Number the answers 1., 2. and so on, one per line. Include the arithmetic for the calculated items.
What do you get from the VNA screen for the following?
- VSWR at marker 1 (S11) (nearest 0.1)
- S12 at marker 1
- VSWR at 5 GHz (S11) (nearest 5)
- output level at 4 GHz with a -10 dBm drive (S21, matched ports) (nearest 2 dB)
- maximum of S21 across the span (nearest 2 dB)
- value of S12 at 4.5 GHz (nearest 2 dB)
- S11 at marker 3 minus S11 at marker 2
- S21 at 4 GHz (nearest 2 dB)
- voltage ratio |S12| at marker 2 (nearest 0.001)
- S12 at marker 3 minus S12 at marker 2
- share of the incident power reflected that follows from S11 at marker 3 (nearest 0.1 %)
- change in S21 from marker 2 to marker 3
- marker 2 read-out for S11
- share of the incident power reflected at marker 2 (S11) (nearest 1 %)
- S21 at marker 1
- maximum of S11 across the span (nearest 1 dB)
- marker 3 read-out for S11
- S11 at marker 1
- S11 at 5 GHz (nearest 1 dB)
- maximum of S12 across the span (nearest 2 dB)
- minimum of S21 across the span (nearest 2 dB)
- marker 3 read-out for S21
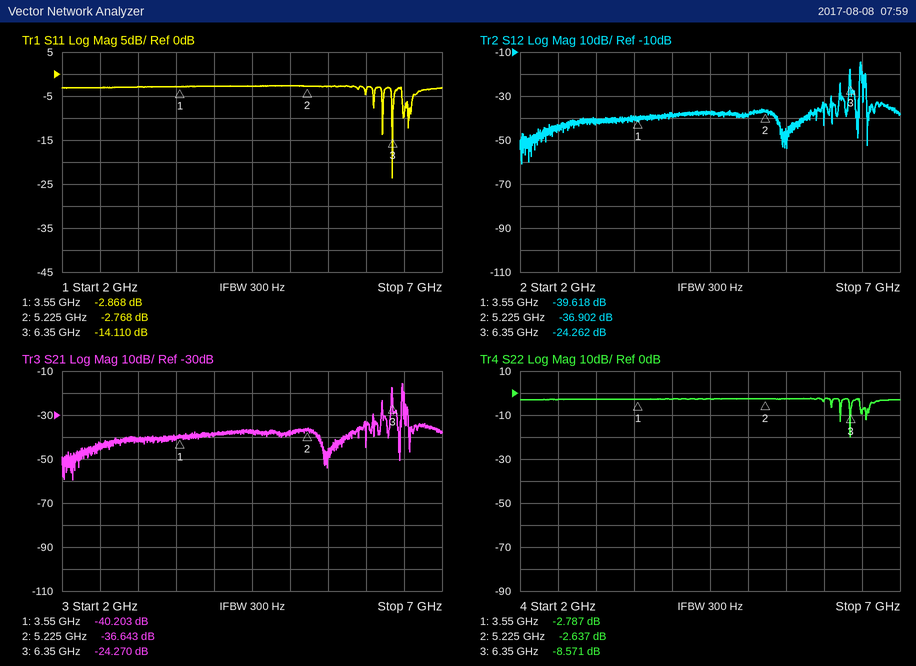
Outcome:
1. (1 + 0.7188)/(1 − 0.7188) ≈ 6.1
2. -39.618 dB
3. |Γ| = 10^(-3/20) = 0.7079; VSWR = (1 + 0.7079)/(1 − 0.7079) ≈ 5.85, so 5 to the nearest 5
4. -10 dBm + (-38 dB) = -48 dBm
5. -16 dB
6. -38 dB
7. -14.11 − (-2.768) = -11.342 dB
8. -38 dB
9. 10^(-36.902/20) ≈ 0.014
10. -24.262 − (-36.902) = 12.640 dB
11. 10^(-14.11/10) ≈ 3.9 %
12. -24.27 − (-36.643) = 12.373 dB
13. -2.768 dB
14. 10^(-2.768/10) ≈ 53 %
15. -40.203 dB
16. -3 dB
17. -14.110 dB
18. -2.868 dB
19. -3 dB
20. -14 dB
21. -60 dB
22. -24.270 dB
